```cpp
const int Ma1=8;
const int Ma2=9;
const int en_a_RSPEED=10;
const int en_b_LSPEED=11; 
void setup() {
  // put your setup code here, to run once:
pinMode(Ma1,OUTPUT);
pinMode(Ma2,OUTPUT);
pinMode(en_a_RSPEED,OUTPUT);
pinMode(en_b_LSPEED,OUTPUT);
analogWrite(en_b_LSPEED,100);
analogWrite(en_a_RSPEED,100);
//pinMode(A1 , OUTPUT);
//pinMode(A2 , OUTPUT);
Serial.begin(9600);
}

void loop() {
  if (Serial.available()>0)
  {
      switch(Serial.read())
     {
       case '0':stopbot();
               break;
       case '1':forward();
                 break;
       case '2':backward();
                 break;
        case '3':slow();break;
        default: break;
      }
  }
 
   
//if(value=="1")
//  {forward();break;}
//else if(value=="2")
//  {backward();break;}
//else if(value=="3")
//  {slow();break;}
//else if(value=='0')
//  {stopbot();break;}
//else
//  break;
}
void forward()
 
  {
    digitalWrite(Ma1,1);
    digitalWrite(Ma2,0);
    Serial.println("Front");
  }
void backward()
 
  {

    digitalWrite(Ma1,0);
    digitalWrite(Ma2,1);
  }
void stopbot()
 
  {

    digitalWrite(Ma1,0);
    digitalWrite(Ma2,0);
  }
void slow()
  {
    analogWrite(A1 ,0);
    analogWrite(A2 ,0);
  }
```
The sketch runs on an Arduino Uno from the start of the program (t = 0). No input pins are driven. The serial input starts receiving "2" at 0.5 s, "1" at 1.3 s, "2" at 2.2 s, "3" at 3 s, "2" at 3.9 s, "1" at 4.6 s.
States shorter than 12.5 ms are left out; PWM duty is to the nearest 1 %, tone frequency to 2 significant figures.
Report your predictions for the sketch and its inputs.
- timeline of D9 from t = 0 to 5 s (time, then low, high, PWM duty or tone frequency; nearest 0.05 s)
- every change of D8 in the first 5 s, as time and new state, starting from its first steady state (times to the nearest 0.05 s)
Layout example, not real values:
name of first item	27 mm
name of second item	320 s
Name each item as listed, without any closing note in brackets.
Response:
timeline of D9 from t = 0 to 5 s	0 s low; 0.5 s high; 1.3 s low; 2.2 s high; 4.6 s low
every change of D8 in the first 5 s, as time and new state, starting from its first steady state	0 s low; 1.3 s high; 2.2 s low; 4.6 s high
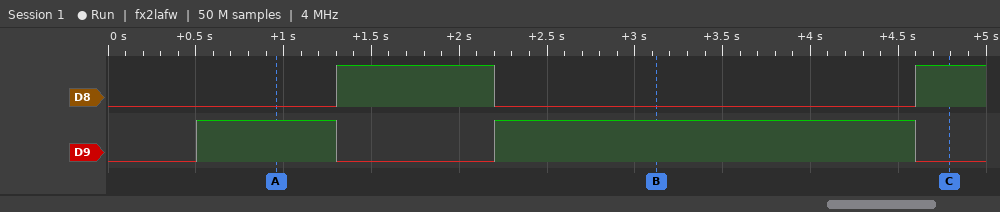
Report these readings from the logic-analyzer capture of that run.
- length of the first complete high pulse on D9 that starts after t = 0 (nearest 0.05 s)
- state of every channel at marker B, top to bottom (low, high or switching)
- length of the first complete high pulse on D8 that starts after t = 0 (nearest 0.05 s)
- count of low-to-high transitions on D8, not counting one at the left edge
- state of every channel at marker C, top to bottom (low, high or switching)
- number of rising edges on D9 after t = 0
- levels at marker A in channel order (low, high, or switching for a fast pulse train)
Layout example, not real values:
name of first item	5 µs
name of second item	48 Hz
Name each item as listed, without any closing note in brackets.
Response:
length of the first complete high pulse on D9 that starts after t = 0	0.80 s
state of every channel at marker B, top to bottom	D8 low, D9 high
length of the first complete high pulse on D8 that starts after t = 0	0.90 s
count of low-to-high transitions on D8, not counting one at the left edge	2
state of every channel at marker C, top to bottom	D8 high, D9 low
number of rising edges on D9 after t = 0	2
levels at marker A in channel order	D8 low, D9 high
